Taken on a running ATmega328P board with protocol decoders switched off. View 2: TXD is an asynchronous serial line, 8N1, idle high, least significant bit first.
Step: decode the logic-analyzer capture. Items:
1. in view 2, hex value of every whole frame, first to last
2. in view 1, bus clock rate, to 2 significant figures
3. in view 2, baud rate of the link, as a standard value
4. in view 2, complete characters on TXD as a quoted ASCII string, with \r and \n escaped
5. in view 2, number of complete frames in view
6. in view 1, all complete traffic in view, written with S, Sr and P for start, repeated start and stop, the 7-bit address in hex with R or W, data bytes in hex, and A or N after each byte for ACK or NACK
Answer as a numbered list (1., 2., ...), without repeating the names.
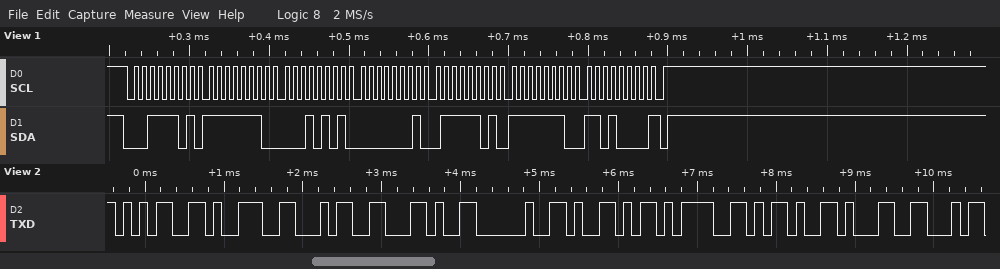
1. 35 39 34 2C 20 59 3D 2D 31
2. 100 kHz
3. 9600 baud
4. "594, Y=-1"
5. 9
6. S 1ER A FE A 15 A 01 A 7D A FE A D0 N P
